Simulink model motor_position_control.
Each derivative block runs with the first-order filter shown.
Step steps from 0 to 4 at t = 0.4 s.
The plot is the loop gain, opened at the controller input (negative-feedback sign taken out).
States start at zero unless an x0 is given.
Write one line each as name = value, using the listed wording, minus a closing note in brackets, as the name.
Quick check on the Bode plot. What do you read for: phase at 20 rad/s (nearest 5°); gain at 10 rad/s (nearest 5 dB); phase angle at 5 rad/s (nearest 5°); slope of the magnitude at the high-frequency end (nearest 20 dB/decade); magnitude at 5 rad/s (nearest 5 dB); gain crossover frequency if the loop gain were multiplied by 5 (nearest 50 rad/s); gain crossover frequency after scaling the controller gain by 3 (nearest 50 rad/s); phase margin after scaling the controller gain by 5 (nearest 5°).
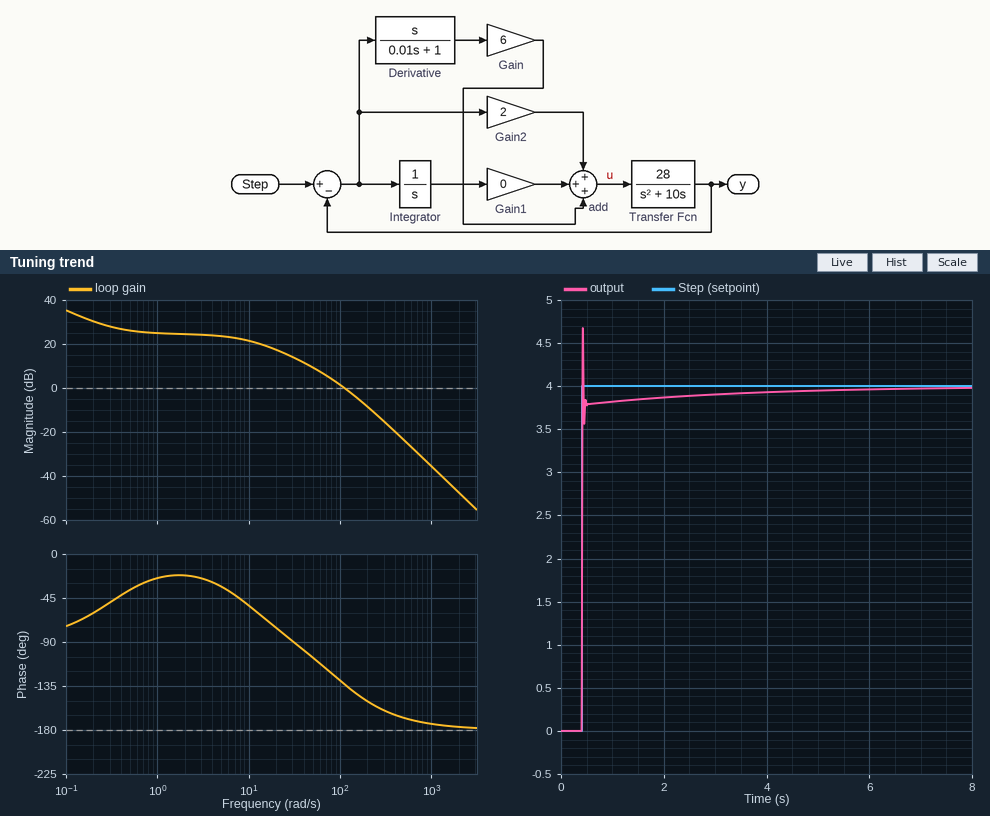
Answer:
phase at 20 rad/s = -75°
gain at 10 rad/s = 20 dB
phase angle at 5 rad/s = -35°
slope of the magnitude at the high-frequency end = -40 dB/decade
magnitude at 5 rad/s = 25 dB
gain crossover frequency if the loop gain were multiplied by 5 = 300 rad/s
gain crossover frequency after scaling the controller gain by 3 = 200 rad/s
phase margin after scaling the controller gain by 5 = 20°
